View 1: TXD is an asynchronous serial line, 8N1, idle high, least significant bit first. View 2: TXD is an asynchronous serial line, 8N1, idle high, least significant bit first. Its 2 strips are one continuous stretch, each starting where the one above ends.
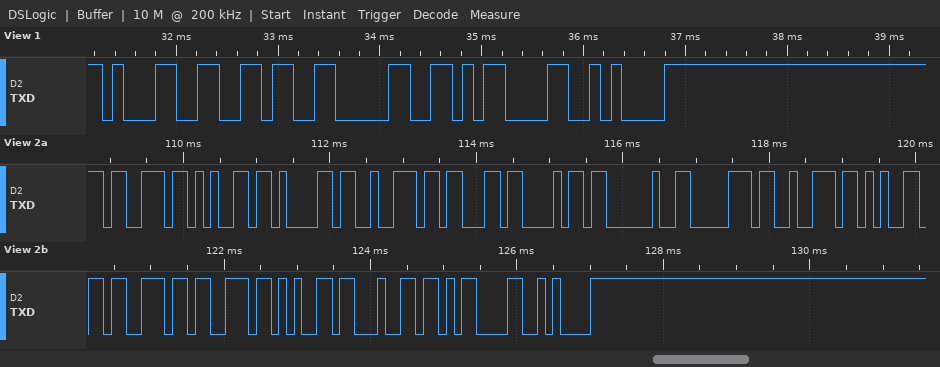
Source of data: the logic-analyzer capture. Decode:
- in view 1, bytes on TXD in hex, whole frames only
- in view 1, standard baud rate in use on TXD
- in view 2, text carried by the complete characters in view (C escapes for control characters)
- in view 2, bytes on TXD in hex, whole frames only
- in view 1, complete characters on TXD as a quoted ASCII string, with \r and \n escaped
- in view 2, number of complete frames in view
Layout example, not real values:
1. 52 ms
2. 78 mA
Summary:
1. 31 36 30 0D 0A
2. 9600 baud
3. "search pressed\r\n"
4. 73 65 61 72 63 68 20 70 72 65 73 73 65 64 0D 0A
5. "160\r\n"
6. 16
